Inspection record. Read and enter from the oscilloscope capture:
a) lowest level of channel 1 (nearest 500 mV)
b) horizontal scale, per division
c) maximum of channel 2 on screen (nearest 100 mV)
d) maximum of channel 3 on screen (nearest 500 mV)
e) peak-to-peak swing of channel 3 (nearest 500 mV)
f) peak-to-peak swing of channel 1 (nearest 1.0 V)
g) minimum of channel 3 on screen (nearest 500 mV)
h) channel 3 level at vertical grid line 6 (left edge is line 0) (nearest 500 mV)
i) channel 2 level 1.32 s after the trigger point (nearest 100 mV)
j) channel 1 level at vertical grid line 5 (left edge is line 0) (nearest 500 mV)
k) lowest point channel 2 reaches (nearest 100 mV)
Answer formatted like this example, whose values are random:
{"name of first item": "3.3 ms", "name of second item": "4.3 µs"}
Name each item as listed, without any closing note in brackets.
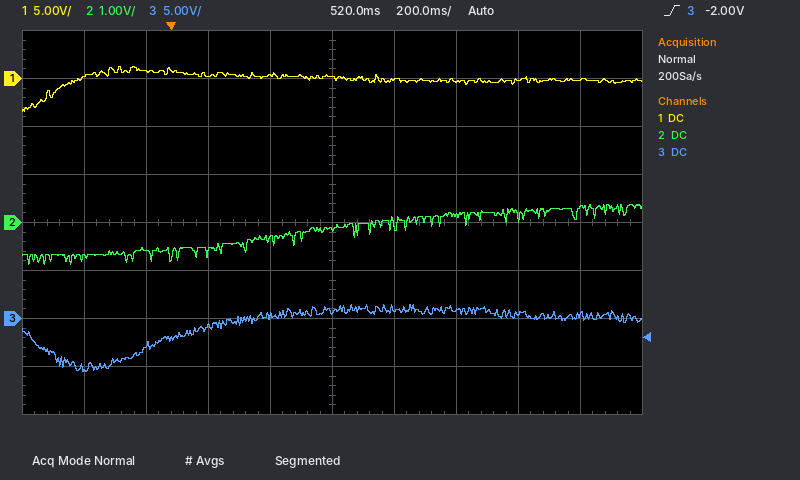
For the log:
{"lowest level of channel 1": "-3.5 V", "horizontal scale, per division": "200 ms", "maximum of channel 2 on screen": "400 mV", "maximum of channel 3 on screen": "1.5 V", "peak-to-peak swing of channel 3": "7.0 V", "peak-to-peak swing of channel 1": "5.0 V", "minimum of channel 3 on screen": "-5.5 V", "channel 3 level at vertical grid line 6 (left edge is line 0)": "1.0 V", "channel 2 level 1.32 s after the trigger point": "300 mV", "channel 1 level at vertical grid line 5 (left edge is line 0)": "0.0 V", "lowest point channel 2 reaches": "-900 mV"}
